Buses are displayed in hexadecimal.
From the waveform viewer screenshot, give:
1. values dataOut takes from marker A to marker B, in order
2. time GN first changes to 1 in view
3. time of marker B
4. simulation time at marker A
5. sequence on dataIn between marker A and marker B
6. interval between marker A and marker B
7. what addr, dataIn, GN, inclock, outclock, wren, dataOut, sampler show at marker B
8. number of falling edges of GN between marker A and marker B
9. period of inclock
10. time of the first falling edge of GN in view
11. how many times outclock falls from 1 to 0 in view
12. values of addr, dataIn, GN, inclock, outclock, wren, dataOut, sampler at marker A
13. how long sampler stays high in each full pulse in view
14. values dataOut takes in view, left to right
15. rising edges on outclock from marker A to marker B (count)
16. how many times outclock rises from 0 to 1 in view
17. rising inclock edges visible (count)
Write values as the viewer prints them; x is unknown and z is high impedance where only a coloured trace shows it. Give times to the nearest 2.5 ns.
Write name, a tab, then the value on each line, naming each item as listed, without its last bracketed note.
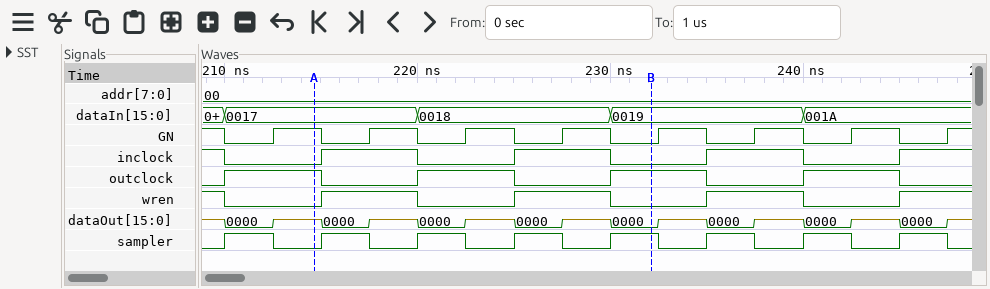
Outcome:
values dataOut takes from marker A to marker B, in order	z, 0000, z, 0000, z, 0000, z, 0000
time GN first changes to 1 in view	212.5 ns
time of marker B	232.5 ns
simulation time at marker A	215 ns
sequence on dataIn between marker A and marker B	0017, 0018, 0019
interval between marker A and marker B	17.5 ns
what addr, dataIn, GN, inclock, outclock, wren, dataOut, sampler show at marker B	addr=00, dataIn=0019, GN=0, inclock=0, outclock=1, wren=0, dataOut=0000, sampler=1
number of falling edges of GN between marker A and marker B	4
period of inclock	10 ns
time of the first falling edge of GN in view	210 ns
how many times outclock falls from 1 to 0 in view	4
values of addr, dataIn, GN, inclock, outclock, wren, dataOut, sampler at marker A	addr=00, dataIn=0017, GN=1, inclock=0, outclock=1, wren=0, dataOut=z, sampler=0
how long sampler stays high in each full pulse in view	2.5 ns, 2.5 ns, 2.5 ns, 2.5 ns, 2.5 ns, 2.5 ns, 2.5 ns, 2.5 ns
values dataOut takes in view, left to right	z, 0000, z, 0000, z, 0000, z, 0000, z, 0000, z, 0000, z, 0000, z, 0000, z
rising edges on outclock from marker A to marker B	2
how many times outclock rises from 0 to 1 in view	4
rising inclock edges visible	4
